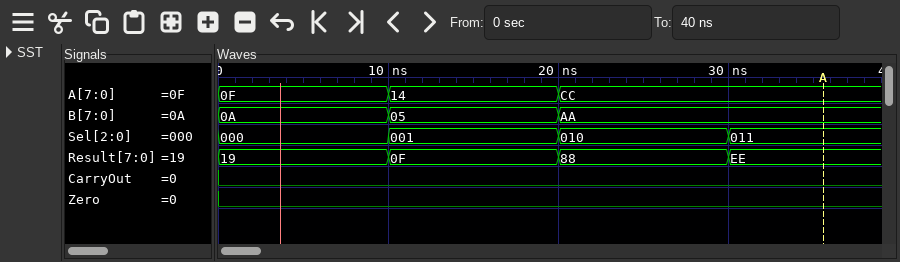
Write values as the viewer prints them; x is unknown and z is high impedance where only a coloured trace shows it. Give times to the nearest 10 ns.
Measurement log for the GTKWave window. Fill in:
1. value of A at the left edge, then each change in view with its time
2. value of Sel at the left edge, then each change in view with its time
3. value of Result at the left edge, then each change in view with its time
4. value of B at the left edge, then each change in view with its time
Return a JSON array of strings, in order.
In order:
["0F, 14 at 10 ns, CC at 20 ns", "000, 001 at 10 ns, 010 at 20 ns, 011 at 30 ns", "19, 0F at 10 ns, 88 at 20 ns, EE at 30 ns", "0A, 05 at 10 ns, AA at 20 ns"]
